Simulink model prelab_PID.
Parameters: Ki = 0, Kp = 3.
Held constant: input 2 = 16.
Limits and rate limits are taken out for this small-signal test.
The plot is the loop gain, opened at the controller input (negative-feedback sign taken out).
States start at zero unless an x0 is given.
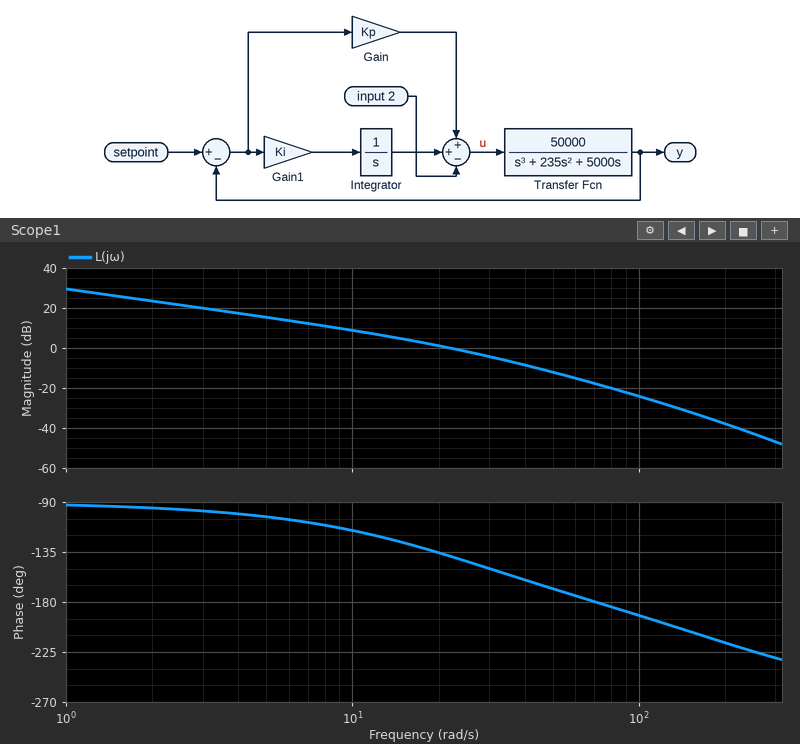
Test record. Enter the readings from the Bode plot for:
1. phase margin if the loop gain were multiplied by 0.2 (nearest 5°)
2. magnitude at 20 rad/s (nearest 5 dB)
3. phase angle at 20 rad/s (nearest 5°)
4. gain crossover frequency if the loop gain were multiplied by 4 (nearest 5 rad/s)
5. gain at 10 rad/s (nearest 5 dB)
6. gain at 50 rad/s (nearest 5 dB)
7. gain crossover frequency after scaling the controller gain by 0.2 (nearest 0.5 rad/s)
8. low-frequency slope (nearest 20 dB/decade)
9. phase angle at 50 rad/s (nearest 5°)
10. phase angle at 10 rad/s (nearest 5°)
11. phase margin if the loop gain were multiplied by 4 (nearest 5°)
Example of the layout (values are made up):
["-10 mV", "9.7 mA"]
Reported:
["75°", "0 dB", "-135°", "50 rad/s", "10 dB", "-10 dB", "6.0 rad/s", "-20 dB/decade", "-170°", "-115°", "10°"]
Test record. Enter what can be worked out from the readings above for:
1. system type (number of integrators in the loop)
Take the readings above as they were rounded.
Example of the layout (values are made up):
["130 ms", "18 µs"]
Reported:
["1"]
